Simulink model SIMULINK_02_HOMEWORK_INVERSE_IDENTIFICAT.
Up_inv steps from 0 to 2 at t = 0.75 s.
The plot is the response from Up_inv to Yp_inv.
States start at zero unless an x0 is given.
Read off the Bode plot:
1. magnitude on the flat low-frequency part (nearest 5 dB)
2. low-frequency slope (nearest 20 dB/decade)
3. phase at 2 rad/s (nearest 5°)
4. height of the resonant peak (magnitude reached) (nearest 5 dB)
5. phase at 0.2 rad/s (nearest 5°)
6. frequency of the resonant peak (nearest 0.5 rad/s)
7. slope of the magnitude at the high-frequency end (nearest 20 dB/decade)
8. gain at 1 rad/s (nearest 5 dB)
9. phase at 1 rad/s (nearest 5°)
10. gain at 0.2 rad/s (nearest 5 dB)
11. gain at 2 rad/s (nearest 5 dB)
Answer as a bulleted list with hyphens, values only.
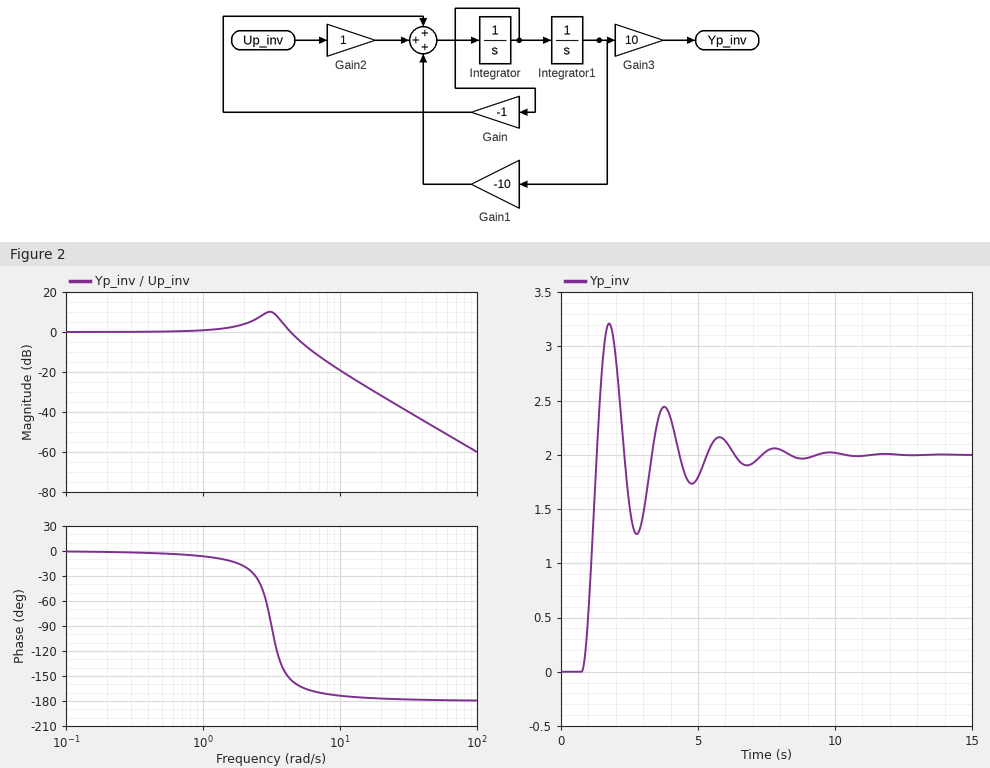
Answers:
- 0 dB
- 0 dB/decade
- -20°
- 10 dB
- 0°
- 3.0 rad/s
- -40 dB/decade
- 0 dB
- -5°
- 0 dB
- 5 dB
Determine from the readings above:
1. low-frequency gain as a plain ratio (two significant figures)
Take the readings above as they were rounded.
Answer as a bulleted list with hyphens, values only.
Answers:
- 1.0
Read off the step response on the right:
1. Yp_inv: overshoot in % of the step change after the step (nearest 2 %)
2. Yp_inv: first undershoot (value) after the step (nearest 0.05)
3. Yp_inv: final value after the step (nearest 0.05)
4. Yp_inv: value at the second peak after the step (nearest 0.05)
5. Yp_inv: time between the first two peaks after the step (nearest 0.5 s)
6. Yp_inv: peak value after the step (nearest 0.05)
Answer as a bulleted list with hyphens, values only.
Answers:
- 60 %
- 1.25
- 2.00
- 2.45
- 2.0 s
- 3.20
